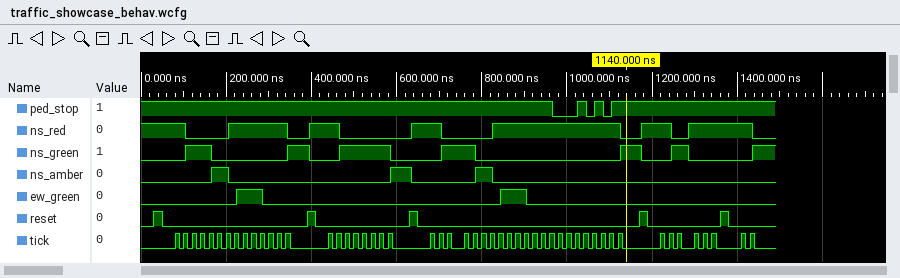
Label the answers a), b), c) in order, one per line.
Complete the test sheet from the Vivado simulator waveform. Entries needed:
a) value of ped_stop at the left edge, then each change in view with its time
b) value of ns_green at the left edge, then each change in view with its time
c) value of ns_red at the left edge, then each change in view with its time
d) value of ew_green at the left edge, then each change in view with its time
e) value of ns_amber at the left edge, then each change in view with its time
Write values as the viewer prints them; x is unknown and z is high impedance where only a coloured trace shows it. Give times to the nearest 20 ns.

a) 1, 0 at 960 ns, 1 at 1020 ns, 0 at 1040 ns, 1 at 1060 ns, 0 at 1080 ns, 1 at 1100 ns
b) 0, 1 at 100 ns, 0 at 160 ns, 1 at 340 ns, 0 at 400 ns, 1 at 460 ns, 0 at 580 ns, 1 at 700 ns, 0 at 780 ns, 1 at 1120 ns, 0 at 1180 ns, 1 at 1240 ns, 0 at 1280 ns, 1 at 1440 ns
c) 1, 0 at 100 ns, 1 at 200 ns, 0 at 340 ns, 1 at 400 ns, 0 at 460 ns, 1 at 640 ns, 0 at 700 ns, 1 at 820 ns, 0 at 1120 ns, 1 at 1180 ns, 0 at 1240 ns, 1 at 1280 ns, 0 at 1440 ns
d) 0, 1 at 220 ns, 0 at 280 ns, 1 at 840 ns, 0 at 900 ns
e) 0, 1 at 160 ns, 0 at 200 ns, 1 at 580 ns, 0 at 640 ns, 1 at 780 ns, 0 at 820 ns
